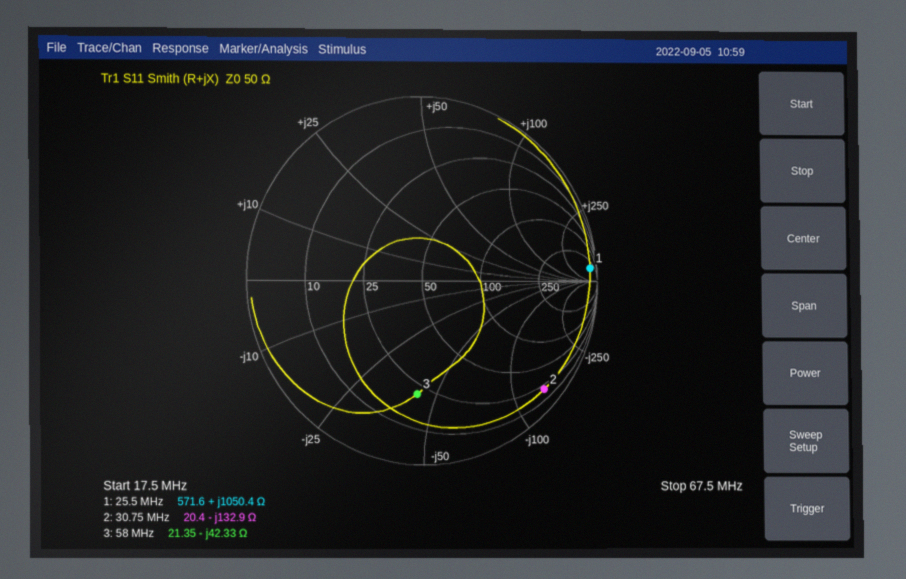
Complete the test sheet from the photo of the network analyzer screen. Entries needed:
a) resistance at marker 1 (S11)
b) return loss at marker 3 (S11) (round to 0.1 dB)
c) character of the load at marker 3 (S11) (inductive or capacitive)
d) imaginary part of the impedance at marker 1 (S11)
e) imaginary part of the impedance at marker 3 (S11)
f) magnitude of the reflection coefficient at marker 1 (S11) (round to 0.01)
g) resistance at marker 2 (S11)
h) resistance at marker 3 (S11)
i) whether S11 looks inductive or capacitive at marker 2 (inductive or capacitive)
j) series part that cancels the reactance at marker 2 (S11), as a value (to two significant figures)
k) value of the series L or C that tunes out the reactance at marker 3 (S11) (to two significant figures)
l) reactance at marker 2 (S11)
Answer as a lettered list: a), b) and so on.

a) 571.6 Ω
b) 4.2 dB
c) capacitive
d) +1050.4 Ω
e) -42.33 Ω
f) 0.96
g) 20.4 Ω
h) 21.35 Ω
i) capacitive
j) 690 nH
k) 120 nH
l) -132.9 Ω
